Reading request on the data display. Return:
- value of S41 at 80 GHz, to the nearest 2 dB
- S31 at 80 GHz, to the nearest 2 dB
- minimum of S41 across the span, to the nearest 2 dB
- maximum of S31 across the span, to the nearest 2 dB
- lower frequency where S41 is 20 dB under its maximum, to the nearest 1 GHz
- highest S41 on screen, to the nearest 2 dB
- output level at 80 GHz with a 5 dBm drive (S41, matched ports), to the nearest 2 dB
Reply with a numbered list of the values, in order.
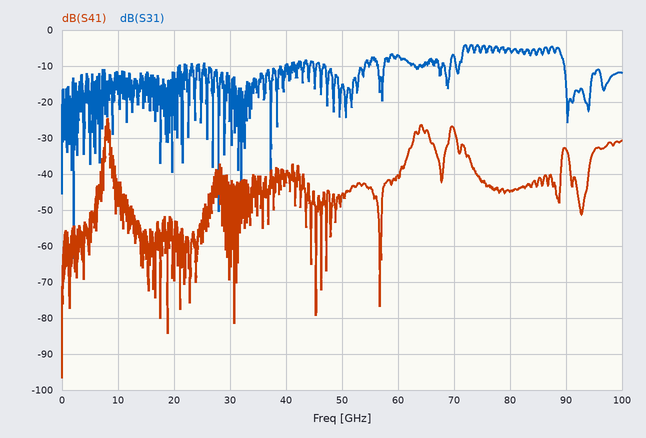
1. -44 dB
2. -6 dB
3. -96 dB
4. -4 dB
5. 7 GHz
6. -24 dB
7. -40 dBm
